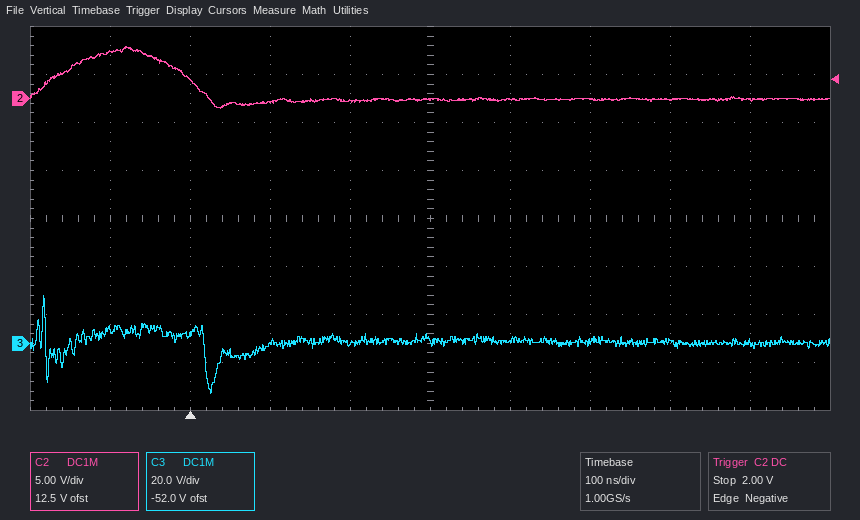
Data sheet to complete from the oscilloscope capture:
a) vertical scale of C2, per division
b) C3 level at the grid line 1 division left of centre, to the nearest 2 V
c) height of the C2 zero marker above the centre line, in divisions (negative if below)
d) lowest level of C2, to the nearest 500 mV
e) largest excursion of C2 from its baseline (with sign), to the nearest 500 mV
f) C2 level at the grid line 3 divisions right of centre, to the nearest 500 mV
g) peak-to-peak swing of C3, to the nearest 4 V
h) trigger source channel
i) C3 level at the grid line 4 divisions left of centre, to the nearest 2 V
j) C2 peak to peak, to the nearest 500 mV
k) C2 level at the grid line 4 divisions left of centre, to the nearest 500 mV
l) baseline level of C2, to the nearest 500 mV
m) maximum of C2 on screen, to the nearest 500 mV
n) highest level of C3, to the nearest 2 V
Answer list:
5 V
0 V
+2.5 div
-1.0 V
+5.5 V
0.0 V
40 V
C2
6 V
6.5 V
5.0 V
0.0 V
5.5 V
20 V
